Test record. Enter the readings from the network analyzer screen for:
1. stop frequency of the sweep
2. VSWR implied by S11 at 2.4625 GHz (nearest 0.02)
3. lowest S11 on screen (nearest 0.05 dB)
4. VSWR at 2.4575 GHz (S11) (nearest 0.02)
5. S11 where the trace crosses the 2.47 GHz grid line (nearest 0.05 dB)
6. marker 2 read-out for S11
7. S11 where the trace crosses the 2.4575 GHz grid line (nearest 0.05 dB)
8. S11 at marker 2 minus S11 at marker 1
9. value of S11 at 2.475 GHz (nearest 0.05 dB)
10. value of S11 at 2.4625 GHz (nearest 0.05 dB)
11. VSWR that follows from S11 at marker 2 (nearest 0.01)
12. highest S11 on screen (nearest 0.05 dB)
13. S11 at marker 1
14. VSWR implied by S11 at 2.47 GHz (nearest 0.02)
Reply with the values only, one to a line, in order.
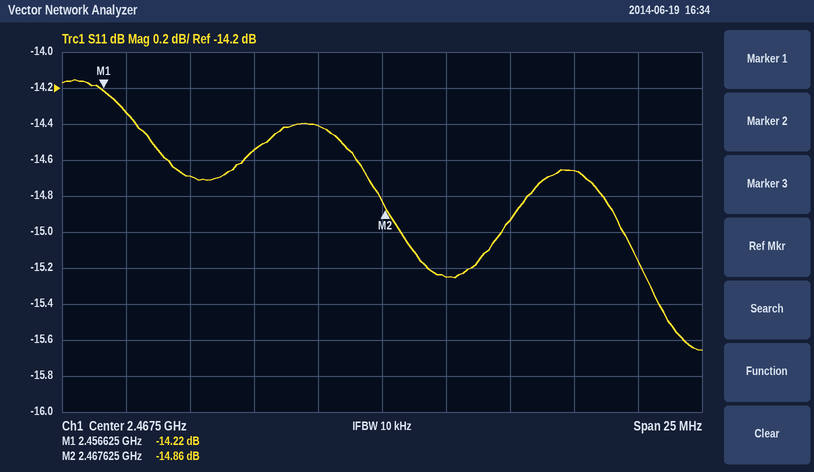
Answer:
2.48 GHz
1.46
-15.65 dB
1.48
-15.25 dB
-14.86 dB
-14.35 dB
-0.64 dB
-14.65 dB
-14.55 dB
1.44
-14.15 dB
-14.22 dB
1.42
